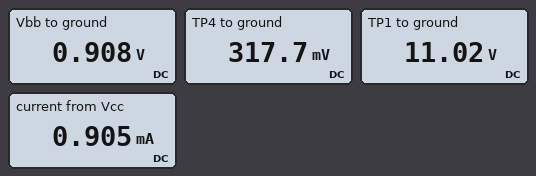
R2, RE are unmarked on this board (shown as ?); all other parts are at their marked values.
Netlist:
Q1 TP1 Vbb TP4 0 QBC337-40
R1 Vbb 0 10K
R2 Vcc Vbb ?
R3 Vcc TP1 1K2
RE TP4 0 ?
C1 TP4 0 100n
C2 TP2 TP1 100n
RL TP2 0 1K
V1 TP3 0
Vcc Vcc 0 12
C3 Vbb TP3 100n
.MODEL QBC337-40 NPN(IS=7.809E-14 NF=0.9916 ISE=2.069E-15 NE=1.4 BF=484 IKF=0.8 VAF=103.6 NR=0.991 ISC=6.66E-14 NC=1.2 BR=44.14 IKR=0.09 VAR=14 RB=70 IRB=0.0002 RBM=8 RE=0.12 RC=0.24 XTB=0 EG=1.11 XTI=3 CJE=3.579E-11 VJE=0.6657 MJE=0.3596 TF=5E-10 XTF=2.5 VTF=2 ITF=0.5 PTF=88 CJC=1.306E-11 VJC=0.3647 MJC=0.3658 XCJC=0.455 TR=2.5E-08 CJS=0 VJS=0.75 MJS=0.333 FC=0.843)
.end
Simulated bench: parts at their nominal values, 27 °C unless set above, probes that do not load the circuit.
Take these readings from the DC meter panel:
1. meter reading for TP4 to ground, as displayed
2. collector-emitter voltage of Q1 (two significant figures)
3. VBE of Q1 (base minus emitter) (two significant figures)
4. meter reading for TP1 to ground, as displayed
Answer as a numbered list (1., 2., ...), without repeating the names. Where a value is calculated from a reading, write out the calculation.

1. 317.7 mV
2. 11.02 V - 317.7 mV = 11 V
3. 908 mV - 317.7 mV = 590 mV
4. 11.02 V
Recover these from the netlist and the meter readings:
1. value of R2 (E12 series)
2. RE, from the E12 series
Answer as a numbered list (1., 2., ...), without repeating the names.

1. 120 kΩ
2. 390 Ω
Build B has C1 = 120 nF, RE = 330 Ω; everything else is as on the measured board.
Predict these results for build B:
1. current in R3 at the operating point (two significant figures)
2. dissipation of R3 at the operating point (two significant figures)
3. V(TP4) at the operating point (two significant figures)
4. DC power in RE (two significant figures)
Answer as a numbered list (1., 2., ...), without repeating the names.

1. 940 µA
2. 1.1 mW
3. 310 mV
4. 290 µW
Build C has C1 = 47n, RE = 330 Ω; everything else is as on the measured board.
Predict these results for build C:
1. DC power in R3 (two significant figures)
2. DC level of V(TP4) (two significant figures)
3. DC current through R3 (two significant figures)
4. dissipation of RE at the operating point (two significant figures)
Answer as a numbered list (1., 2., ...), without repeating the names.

1. 1.1 mW
2. 310 mV
3. 940 µA
4. 290 µW
